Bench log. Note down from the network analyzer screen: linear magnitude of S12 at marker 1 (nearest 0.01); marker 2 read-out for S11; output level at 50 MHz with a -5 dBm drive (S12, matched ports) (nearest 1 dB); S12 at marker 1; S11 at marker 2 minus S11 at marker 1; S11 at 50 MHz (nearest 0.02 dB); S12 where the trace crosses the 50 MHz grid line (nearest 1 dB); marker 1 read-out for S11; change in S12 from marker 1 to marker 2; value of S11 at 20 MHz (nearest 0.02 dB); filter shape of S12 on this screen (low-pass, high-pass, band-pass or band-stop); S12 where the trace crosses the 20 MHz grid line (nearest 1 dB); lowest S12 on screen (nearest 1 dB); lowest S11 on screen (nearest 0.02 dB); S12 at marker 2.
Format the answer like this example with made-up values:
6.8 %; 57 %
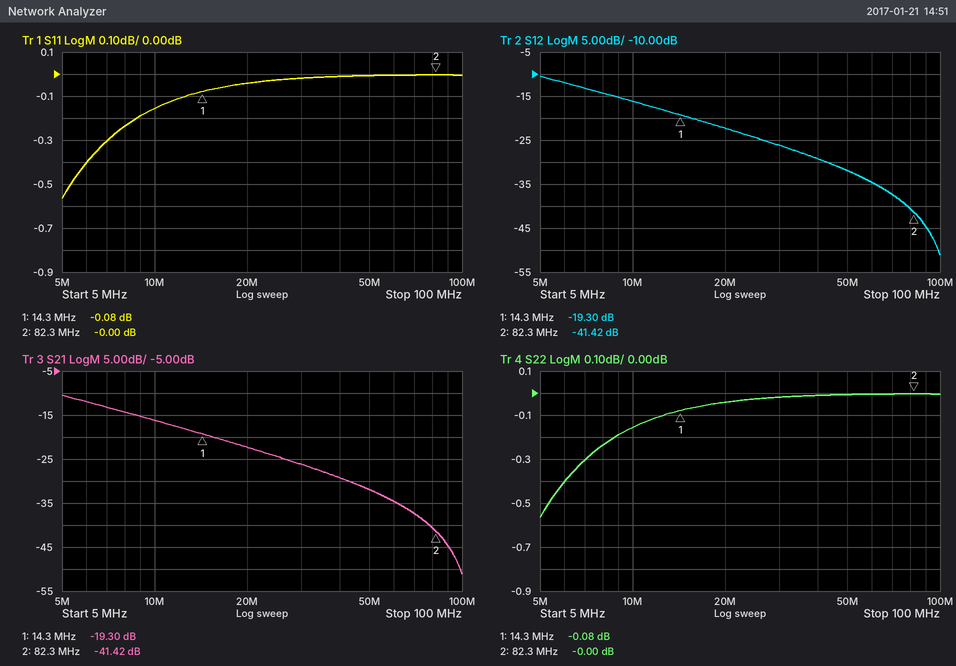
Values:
0.11; -0.00 dB; -37 dBm; -19.30 dB; 0.08 dB; 0.00 dB; -32 dB; -0.08 dB; -22.12 dB; -0.04 dB; low-pass; -22 dB; -51 dB; -0.56 dB; -41.42 dB
